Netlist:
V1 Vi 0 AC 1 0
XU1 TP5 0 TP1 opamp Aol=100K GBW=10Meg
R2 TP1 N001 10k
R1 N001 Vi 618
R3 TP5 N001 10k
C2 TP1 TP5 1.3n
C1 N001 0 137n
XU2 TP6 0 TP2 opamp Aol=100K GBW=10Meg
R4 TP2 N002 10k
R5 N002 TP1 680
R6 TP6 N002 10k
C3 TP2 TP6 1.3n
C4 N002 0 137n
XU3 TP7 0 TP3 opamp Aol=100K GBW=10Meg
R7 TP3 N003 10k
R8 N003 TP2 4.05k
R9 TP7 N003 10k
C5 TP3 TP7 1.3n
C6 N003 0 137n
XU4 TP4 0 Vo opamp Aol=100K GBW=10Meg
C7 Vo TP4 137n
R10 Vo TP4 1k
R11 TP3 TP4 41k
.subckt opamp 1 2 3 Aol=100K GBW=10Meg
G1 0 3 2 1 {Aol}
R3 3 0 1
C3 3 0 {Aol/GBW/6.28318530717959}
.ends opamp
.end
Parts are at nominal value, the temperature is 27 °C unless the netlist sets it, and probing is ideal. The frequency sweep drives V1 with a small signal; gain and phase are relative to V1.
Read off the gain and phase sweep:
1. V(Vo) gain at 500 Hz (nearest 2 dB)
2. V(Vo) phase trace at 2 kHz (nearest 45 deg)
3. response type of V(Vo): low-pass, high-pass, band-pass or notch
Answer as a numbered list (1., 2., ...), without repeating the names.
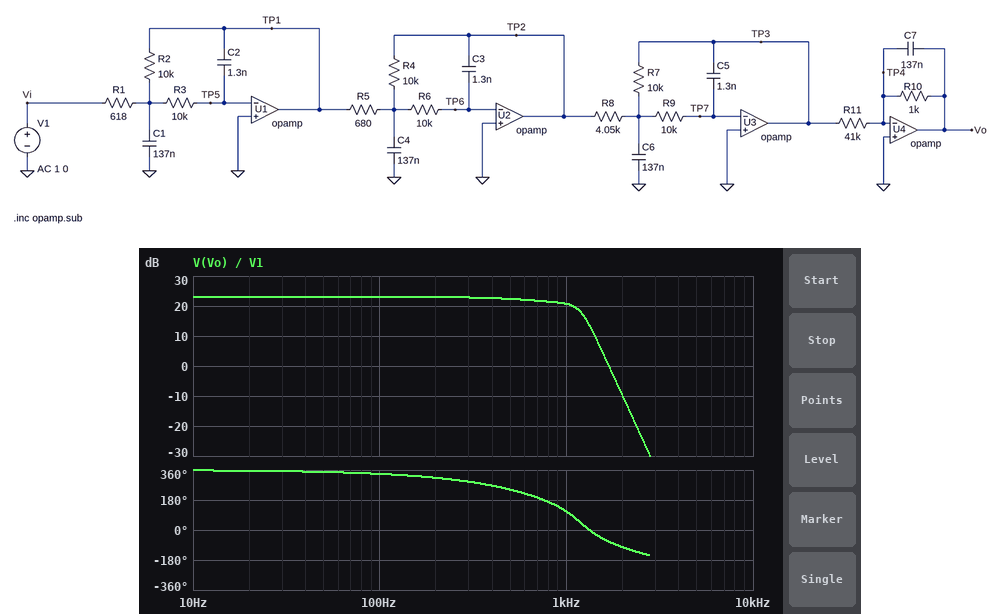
1. 22 dB
2. -90 deg
3. low-pass
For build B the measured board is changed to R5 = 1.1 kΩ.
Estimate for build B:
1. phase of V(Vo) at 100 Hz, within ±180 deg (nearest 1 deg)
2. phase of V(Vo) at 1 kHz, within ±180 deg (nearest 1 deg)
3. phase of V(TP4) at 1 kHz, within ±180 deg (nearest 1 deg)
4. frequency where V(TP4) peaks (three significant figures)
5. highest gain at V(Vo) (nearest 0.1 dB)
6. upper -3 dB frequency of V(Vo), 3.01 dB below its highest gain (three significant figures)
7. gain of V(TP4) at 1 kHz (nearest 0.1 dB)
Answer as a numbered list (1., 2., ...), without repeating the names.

1. -21 deg
2. 118 deg
3. 22 deg
4. 1.06 kHz
5. 20.0 dB
6. 1.21 kHz
7. -60.1 dB
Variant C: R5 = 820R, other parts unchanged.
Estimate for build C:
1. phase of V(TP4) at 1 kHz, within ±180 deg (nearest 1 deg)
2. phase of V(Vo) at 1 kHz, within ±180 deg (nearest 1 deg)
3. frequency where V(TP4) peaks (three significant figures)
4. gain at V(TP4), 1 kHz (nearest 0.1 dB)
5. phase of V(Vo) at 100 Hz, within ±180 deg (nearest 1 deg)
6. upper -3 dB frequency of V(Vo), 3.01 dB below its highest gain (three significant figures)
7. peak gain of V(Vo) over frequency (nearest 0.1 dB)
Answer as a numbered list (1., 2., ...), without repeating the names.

1. 18 deg
2. 114 deg
3. 1.05 kHz
4. -59.5 dB
5. -22 deg
6. 1.16 kHz
7. 21.5 dB
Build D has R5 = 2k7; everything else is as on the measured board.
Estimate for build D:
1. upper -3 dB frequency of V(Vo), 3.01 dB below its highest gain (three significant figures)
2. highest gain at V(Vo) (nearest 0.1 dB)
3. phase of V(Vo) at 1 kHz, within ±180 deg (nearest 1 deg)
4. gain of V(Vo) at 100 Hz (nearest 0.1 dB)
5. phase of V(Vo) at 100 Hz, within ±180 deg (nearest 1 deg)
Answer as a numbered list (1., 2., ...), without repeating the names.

1. 1.24 kHz
2. 17.0 dB
3. 132 deg
4. 11.2 dB
5. -18 deg
